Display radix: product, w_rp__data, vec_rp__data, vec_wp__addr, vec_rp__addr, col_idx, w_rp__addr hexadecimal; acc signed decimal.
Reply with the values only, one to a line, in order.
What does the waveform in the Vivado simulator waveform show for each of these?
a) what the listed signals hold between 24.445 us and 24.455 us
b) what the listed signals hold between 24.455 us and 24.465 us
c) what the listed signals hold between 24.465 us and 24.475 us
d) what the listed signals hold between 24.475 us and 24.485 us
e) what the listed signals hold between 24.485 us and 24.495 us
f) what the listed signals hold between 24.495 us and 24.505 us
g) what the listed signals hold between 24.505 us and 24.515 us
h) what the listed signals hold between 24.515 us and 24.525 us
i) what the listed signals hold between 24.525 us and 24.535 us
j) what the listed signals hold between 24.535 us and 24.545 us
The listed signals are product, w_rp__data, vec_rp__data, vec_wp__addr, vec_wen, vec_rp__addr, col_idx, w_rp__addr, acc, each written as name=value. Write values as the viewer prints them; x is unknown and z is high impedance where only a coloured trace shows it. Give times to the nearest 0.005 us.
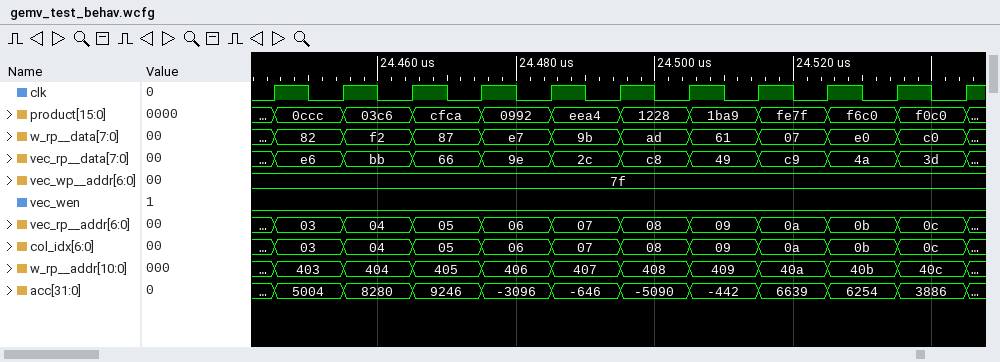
product=0ccc, w_rp__data=82, vec_rp__data=e6, vec_wp__addr=7f, vec_wen=0, vec_rp__addr=03, col_idx=03, w_rp__addr=403, acc=5004
product=03c6, w_rp__data=f2, vec_rp__data=bb, vec_wp__addr=7f, vec_wen=0, vec_rp__addr=04, col_idx=04, w_rp__addr=404, acc=8280
product=cfca, w_rp__data=87, vec_rp__data=66, vec_wp__addr=7f, vec_wen=0, vec_rp__addr=05, col_idx=05, w_rp__addr=405, acc=9246
product=0992, w_rp__data=e7, vec_rp__data=9e, vec_wp__addr=7f, vec_wen=0, vec_rp__addr=06, col_idx=06, w_rp__addr=406, acc=-3096
product=eea4, w_rp__data=9b, vec_rp__data=2c, vec_wp__addr=7f, vec_wen=0, vec_rp__addr=07, col_idx=07, w_rp__addr=407, acc=-646
product=1228, w_rp__data=ad, vec_rp__data=c8, vec_wp__addr=7f, vec_wen=0, vec_rp__addr=08, col_idx=08, w_rp__addr=408, acc=-5090
product=1ba9, w_rp__data=61, vec_rp__data=49, vec_wp__addr=7f, vec_wen=0, vec_rp__addr=09, col_idx=09, w_rp__addr=409, acc=-442
product=fe7f, w_rp__data=07, vec_rp__data=c9, vec_wp__addr=7f, vec_wen=0, vec_rp__addr=0a, col_idx=0a, w_rp__addr=40a, acc=6639
product=f6c0, w_rp__data=e0, vec_rp__data=4a, vec_wp__addr=7f, vec_wen=0, vec_rp__addr=0b, col_idx=0b, w_rp__addr=40b, acc=6254
product=f0c0, w_rp__data=c0, vec_rp__data=3d, vec_wp__addr=7f, vec_wen=0, vec_rp__addr=0c, col_idx=0c, w_rp__addr=40c, acc=3886
